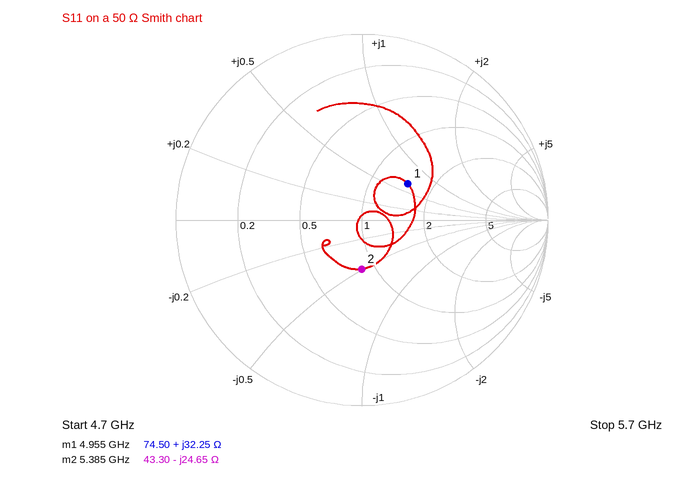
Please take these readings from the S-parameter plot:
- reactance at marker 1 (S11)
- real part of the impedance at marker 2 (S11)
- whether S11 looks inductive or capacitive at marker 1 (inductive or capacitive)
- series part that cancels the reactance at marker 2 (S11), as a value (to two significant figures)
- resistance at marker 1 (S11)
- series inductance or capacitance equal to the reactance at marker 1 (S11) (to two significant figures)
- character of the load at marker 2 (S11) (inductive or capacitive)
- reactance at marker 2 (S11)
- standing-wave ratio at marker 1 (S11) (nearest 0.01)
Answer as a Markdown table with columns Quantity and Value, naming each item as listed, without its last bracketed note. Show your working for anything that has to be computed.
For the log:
| Quantity | Value |
|---|---|
| reactance at marker 1 | +32.25 Ω |
| real part of the impedance at marker 2 | 43.30 Ω |
| whether S11 looks inductive or capacitive at marker 1 | inductive |
| series part that cancels the reactance at marker 2 (S11), as a value | L = 24.65 Ω/(2π × 5.385 GHz) ≈ 729 pH, so 730 pH to two significant figures |
| resistance at marker 1 | 74.50 Ω |
| series inductance or capacitance equal to the reactance at marker 1 (S11) | L = 32.25 Ω/(2π × 4.955 GHz) ≈ 1.0 nH |
| character of the load at marker 2 (S11) | capacitive |
| reactance at marker 2 | -24.65 Ω |
| standing-wave ratio at marker 1 (S11) | 1.92 |
